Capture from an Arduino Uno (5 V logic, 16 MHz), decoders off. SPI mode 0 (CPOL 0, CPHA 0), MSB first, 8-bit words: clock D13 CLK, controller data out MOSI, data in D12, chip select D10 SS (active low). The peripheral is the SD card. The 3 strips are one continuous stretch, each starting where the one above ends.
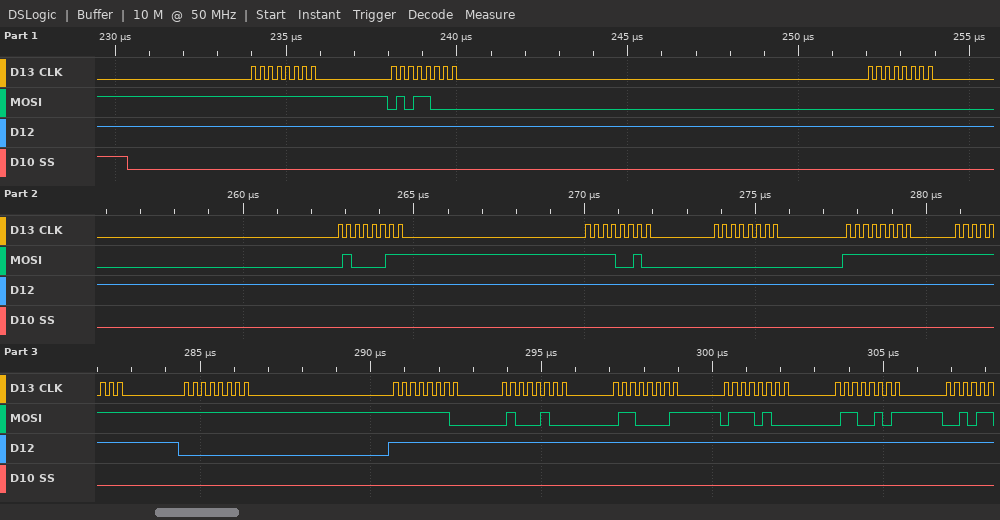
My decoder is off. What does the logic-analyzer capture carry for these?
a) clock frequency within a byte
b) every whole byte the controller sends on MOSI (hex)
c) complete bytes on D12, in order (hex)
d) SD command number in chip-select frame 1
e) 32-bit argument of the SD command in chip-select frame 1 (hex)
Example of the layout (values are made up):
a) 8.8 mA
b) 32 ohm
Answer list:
a) 4 MHz
b) 0xFF 0x58 0x00 0x43 0xF2 0x00 0xFF 0xFF 0xFF 0xFE 0x44 0x61 0x74 0x65
c) 0xFF 0xFF 0xFF 0xFF 0xFF 0xFF 0xFF 0xFF 0x00 0xFF 0xFF 0xFF 0xFF 0xFF
d) CMD24
e) 0x0043F200
